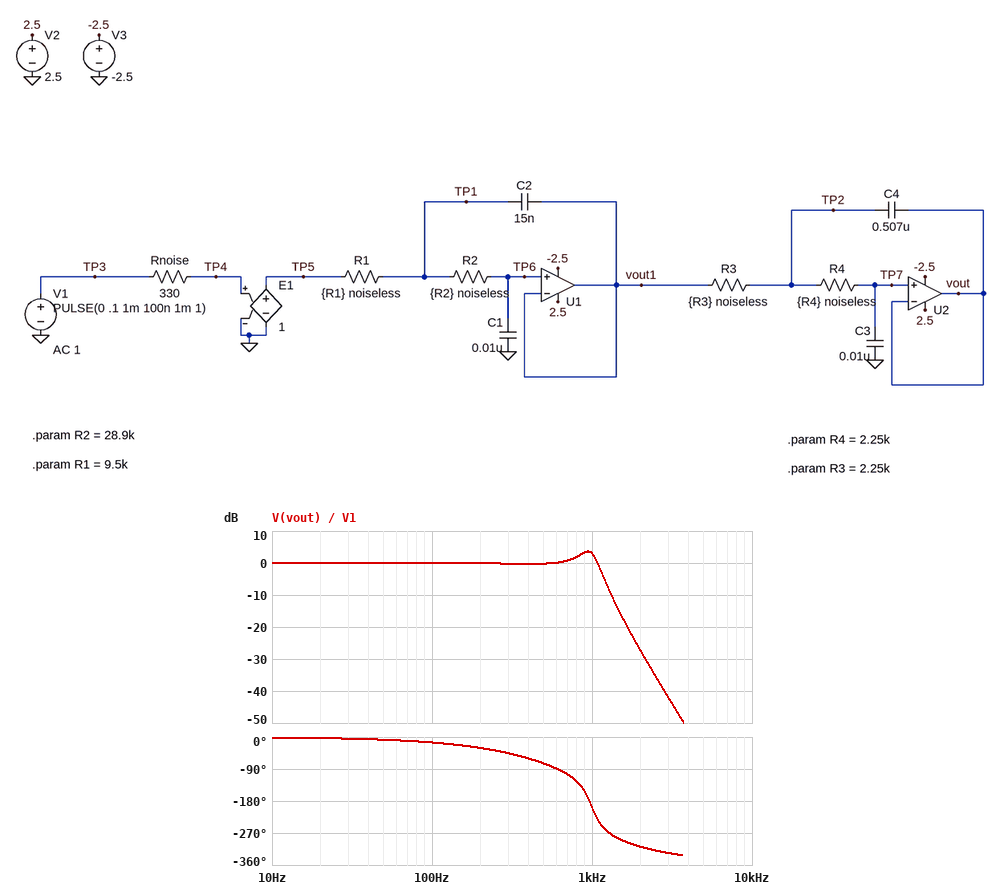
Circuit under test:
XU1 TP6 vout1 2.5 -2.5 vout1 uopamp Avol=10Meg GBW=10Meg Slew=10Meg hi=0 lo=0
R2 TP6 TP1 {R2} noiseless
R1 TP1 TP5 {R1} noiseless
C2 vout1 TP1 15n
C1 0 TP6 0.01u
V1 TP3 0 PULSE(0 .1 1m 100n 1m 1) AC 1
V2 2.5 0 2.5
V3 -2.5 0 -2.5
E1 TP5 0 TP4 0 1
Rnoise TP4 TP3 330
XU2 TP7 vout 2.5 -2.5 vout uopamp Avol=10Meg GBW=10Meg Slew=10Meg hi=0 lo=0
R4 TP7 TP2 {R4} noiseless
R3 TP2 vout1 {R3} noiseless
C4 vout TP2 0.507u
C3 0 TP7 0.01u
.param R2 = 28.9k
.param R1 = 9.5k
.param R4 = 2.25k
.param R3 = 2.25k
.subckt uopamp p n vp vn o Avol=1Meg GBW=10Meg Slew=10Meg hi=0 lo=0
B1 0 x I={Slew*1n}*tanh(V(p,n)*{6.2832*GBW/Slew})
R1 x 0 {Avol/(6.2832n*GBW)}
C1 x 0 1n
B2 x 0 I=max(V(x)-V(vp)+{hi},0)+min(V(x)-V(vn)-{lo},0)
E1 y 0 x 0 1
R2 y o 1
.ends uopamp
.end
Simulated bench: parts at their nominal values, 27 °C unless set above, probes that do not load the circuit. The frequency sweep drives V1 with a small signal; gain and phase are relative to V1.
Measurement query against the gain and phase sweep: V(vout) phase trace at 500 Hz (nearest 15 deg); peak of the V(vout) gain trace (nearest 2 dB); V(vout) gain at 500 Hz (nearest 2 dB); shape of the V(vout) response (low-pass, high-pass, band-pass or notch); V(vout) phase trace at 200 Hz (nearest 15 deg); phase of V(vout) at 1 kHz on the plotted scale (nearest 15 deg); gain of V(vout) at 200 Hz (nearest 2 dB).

-75 deg
4 dB
0 dB
low-pass
-30 deg
-195 deg
0 dB
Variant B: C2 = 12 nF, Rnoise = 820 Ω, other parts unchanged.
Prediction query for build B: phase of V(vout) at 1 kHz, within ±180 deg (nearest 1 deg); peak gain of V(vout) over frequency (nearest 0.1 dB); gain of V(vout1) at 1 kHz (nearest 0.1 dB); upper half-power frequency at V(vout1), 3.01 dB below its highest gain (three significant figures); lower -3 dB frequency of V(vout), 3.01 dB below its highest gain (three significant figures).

170 deg
3.8 dB
-7.7 dB
521 Hz
717 Hz
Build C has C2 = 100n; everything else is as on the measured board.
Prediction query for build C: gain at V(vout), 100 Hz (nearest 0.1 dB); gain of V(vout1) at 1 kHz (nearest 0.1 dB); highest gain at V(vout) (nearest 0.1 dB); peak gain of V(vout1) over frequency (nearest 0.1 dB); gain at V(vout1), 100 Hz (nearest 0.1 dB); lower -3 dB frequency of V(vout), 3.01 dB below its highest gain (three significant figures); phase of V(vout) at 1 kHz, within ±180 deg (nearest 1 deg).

0.8 dB
-20.1 dB
3.9 dB
3.3 dB
0.7 dB
109 Hz
101 deg
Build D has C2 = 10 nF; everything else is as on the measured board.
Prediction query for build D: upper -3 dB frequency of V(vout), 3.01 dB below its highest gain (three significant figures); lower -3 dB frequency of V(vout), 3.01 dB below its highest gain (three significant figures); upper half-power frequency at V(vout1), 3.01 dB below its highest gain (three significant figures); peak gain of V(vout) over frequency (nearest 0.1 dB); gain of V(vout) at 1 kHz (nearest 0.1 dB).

1.08 kHz
730 Hz
503 Hz
3.8 dB
3.3 dB
